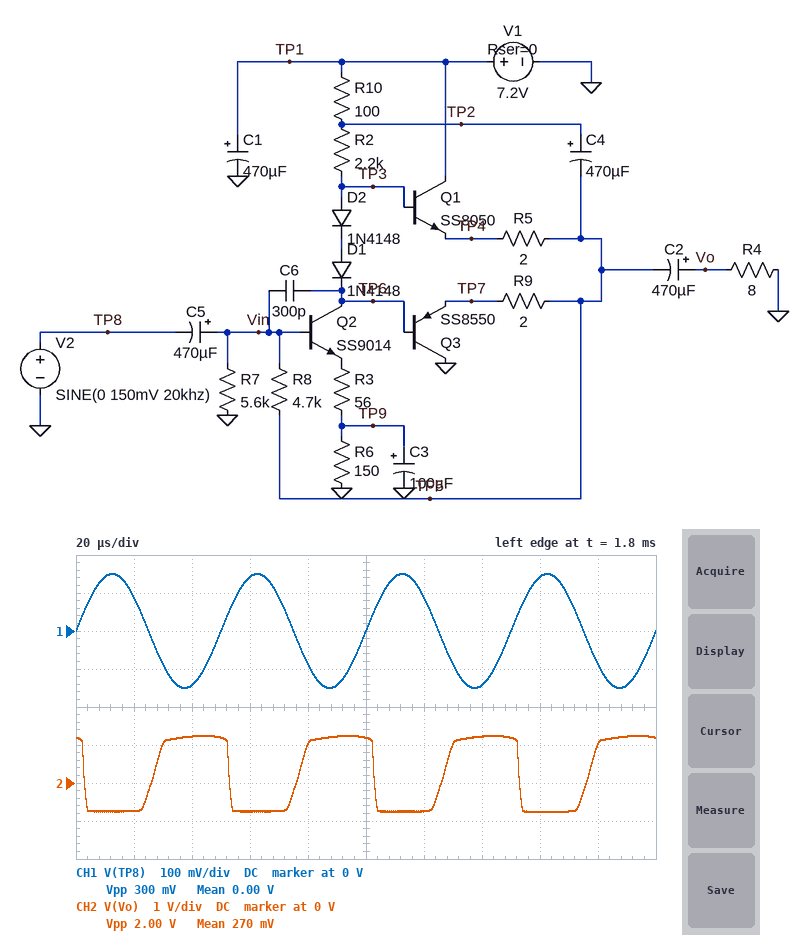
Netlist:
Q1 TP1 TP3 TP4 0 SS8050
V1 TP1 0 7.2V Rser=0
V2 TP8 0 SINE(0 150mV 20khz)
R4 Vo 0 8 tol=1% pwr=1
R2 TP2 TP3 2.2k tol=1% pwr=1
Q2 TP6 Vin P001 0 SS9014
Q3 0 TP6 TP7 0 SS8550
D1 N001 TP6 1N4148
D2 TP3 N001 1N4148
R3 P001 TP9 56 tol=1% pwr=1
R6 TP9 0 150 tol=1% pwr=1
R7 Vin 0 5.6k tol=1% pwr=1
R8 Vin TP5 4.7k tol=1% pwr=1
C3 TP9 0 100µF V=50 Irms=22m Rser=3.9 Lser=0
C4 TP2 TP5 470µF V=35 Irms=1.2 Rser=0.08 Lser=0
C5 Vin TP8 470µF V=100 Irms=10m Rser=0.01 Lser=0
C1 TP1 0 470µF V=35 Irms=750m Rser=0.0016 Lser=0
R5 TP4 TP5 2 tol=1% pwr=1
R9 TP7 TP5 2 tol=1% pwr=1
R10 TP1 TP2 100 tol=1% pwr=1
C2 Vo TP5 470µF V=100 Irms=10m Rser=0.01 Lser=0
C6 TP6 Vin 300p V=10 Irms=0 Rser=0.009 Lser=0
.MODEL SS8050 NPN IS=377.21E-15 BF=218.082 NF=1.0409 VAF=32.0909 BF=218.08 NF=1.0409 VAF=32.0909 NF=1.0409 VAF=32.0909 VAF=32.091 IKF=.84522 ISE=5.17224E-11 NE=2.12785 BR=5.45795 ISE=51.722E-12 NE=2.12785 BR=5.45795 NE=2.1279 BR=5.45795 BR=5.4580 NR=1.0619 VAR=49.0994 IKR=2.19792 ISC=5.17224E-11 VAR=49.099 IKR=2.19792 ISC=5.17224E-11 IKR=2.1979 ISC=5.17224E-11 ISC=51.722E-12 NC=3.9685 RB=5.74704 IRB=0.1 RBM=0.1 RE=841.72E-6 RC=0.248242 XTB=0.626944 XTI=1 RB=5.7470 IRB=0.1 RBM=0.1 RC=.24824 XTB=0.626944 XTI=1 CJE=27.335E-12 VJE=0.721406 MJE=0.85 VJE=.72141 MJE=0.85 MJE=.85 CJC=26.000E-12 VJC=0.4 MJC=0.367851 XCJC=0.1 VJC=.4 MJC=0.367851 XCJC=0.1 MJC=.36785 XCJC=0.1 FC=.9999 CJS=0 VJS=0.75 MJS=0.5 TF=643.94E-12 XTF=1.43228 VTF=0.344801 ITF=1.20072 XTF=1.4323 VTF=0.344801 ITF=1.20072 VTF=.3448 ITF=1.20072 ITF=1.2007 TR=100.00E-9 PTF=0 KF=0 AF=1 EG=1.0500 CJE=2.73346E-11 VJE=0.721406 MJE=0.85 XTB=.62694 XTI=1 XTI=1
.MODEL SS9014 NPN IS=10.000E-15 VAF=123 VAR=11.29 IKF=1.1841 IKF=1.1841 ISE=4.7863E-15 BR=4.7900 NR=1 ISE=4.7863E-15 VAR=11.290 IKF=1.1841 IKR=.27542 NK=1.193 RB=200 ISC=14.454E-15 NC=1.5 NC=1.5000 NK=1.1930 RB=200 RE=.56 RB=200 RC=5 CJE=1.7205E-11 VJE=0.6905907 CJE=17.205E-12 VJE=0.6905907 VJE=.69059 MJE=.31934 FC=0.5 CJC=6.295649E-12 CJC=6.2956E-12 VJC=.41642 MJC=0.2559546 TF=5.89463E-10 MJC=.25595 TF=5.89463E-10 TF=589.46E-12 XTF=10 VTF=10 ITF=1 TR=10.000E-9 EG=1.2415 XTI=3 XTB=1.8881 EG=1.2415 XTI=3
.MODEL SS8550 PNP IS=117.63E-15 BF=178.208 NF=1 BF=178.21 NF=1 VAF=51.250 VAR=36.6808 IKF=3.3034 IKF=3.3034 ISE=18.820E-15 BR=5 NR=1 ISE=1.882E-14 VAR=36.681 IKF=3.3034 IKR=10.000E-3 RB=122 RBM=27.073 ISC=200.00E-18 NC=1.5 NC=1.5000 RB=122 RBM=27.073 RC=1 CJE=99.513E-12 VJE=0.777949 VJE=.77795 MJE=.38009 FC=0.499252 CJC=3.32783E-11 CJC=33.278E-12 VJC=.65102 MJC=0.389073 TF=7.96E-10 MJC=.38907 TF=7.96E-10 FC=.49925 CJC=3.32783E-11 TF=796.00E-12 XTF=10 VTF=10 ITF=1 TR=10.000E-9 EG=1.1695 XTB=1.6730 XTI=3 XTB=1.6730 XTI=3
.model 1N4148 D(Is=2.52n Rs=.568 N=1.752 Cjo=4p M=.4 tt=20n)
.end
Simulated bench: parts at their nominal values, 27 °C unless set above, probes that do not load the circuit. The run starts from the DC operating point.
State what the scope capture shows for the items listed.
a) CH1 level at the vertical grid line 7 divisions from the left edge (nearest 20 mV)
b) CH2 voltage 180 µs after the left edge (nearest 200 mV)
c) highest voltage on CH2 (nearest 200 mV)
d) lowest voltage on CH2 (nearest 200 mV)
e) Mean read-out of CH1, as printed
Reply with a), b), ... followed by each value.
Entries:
a) -140 mV
b) 1.0 V
c) 1.2 V
d) -800 mV
e) 0.00 V
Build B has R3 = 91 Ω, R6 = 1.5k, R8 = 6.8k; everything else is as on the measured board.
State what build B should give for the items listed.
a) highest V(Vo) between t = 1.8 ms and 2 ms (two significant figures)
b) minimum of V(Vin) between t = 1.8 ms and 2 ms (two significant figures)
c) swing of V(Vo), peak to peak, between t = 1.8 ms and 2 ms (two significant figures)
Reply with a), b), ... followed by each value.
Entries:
a) 890 mV
b) 1.9 V
c) 2.2 V
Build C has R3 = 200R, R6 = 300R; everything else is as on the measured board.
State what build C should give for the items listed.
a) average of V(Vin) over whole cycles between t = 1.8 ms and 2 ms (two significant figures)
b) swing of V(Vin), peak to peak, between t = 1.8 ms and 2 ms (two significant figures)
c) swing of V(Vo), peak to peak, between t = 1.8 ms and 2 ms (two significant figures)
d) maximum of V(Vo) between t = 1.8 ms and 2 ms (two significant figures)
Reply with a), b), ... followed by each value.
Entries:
a) 1.5 V
b) 300 mV
c) 1.4 V
d) 760 mV
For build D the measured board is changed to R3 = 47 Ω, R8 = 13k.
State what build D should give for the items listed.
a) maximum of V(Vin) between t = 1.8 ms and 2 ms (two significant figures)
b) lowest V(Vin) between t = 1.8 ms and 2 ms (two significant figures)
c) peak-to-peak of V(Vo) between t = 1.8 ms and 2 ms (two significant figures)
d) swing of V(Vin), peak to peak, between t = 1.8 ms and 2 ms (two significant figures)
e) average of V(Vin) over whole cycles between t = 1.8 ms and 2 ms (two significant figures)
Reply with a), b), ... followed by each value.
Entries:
a) 1.1 V
b) 800 mV
c) 2.8 V
d) 300 mV
e) 950 mV
